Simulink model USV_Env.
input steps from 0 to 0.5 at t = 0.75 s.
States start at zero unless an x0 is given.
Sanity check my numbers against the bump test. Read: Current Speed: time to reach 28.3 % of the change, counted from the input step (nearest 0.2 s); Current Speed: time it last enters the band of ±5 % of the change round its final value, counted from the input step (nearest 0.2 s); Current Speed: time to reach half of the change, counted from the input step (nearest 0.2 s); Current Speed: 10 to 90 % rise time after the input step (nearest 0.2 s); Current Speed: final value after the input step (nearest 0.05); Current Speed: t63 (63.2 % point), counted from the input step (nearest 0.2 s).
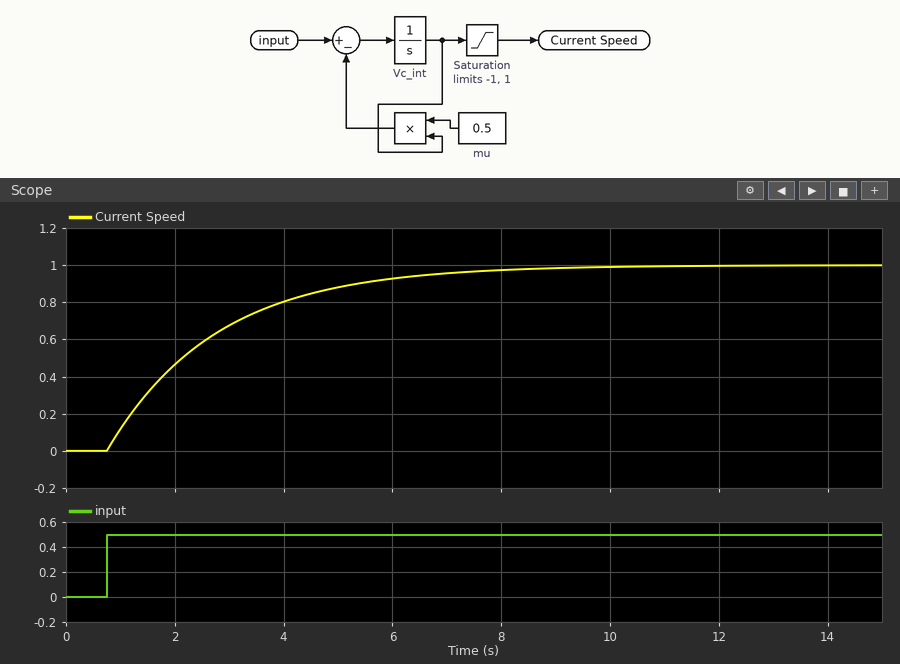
0.6 s
6.0 s
1.4 s
4.4 s
1.00
2.0 s
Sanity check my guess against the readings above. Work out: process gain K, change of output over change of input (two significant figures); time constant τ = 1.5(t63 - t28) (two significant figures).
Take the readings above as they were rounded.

2.0
2.1 s
